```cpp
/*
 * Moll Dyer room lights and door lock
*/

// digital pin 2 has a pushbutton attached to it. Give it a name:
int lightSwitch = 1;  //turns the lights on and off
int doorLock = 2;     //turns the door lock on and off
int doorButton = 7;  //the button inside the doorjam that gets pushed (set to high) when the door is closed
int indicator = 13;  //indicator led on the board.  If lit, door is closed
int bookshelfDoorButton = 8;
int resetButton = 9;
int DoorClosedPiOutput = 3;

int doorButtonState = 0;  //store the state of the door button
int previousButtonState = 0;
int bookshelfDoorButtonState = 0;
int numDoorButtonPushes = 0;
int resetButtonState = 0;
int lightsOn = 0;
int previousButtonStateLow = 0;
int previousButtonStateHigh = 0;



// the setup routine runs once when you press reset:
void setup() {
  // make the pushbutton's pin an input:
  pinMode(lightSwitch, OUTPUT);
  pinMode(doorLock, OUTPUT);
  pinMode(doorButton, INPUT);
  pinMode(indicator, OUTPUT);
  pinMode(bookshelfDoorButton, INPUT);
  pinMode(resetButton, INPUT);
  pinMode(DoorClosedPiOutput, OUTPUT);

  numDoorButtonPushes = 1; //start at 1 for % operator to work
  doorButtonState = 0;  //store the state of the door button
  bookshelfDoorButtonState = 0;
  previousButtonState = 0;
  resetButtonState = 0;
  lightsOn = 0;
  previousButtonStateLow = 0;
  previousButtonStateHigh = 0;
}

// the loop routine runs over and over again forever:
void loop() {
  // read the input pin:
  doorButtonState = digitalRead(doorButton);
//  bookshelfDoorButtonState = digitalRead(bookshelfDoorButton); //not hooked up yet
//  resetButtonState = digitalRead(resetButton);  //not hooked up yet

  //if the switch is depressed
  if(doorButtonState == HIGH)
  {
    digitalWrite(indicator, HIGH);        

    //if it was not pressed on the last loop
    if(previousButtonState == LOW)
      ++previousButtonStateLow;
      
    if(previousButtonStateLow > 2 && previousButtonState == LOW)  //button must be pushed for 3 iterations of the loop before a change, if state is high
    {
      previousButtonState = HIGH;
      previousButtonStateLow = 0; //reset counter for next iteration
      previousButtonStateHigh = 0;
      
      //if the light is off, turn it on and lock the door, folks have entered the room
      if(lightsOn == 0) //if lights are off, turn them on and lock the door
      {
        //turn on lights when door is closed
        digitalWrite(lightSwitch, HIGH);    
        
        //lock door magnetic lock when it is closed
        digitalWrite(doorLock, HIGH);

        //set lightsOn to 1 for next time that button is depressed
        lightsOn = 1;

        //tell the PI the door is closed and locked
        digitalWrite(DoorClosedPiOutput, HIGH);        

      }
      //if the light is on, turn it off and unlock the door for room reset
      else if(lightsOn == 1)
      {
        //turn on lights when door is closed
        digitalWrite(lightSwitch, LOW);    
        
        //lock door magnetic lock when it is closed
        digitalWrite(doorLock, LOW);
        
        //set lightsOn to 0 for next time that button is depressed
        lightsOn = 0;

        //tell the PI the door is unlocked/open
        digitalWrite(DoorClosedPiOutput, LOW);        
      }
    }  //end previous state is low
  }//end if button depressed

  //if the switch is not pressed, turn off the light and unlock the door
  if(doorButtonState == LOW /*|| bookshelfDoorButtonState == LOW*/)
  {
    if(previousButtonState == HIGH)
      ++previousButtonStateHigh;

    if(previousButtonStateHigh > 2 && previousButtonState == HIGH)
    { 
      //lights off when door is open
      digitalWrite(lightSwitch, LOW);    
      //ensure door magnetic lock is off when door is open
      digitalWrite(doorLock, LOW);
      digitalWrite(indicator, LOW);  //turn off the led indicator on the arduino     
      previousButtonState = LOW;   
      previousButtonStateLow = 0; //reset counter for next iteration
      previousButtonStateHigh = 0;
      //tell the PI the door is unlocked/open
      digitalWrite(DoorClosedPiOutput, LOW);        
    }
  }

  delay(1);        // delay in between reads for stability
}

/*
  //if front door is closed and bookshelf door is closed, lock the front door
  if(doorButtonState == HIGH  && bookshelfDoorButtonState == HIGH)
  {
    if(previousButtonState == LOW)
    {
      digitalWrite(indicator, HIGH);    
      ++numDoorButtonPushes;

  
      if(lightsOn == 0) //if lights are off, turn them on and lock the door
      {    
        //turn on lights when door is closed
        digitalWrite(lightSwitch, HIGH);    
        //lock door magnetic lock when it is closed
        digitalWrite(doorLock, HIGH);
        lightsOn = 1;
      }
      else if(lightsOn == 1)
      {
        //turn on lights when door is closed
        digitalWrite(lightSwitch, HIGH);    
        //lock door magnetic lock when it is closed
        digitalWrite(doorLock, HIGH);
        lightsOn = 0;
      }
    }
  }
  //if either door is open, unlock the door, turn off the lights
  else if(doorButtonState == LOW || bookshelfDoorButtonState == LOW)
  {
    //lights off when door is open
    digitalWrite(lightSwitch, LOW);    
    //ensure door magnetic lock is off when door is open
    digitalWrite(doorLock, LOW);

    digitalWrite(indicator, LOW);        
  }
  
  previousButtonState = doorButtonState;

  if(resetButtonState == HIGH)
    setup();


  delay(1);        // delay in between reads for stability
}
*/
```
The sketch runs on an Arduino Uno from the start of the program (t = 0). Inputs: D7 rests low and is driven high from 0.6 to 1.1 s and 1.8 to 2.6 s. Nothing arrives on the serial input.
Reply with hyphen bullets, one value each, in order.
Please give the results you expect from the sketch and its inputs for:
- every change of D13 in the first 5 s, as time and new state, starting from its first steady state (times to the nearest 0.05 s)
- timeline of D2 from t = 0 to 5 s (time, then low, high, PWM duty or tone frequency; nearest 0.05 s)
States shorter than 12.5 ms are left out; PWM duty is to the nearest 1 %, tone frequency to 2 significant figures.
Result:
- 0 s low; 0.6 s high; 1.1 s low; 1.8 s high; 2.6 s low
- 0 s low; 0.6 s high; 1.1 s low
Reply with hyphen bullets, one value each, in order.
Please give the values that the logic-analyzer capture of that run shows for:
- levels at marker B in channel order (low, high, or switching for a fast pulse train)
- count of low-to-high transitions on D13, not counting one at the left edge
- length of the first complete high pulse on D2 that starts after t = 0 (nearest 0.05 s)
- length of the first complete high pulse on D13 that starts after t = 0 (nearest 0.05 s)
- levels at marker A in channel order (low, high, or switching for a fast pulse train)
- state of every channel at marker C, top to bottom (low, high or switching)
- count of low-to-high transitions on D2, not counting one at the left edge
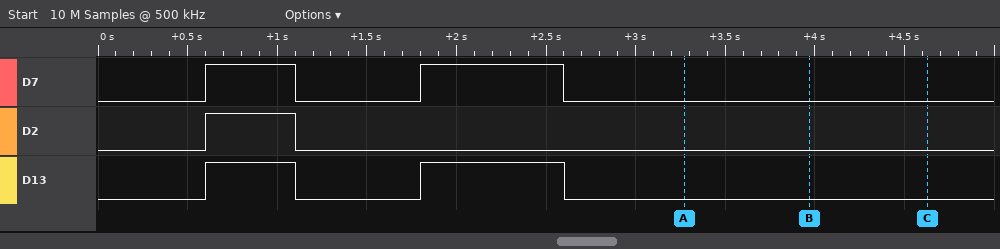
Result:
- D7 low, D2 low, D13 low
- 2
- 0.50 s
- 0.50 s
- D7 low, D2 low, D13 low
- D7 low, D2 low, D13 low
- 1
